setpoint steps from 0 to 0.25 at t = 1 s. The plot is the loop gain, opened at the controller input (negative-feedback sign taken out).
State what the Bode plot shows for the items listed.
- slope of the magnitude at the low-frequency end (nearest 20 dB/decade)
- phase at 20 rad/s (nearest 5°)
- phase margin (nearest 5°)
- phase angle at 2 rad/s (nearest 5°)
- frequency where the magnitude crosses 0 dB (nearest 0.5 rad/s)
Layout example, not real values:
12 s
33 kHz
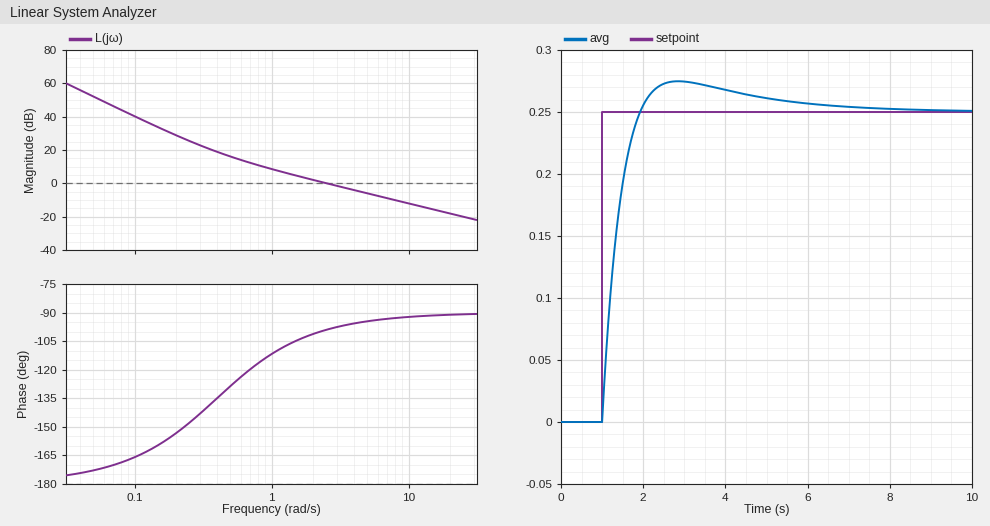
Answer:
-40 dB/decade
-90°
80°
-100°
2.5 rad/s
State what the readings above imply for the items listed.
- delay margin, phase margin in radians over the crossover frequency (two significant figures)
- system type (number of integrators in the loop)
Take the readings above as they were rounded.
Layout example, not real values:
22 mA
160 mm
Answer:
0.56 s
2
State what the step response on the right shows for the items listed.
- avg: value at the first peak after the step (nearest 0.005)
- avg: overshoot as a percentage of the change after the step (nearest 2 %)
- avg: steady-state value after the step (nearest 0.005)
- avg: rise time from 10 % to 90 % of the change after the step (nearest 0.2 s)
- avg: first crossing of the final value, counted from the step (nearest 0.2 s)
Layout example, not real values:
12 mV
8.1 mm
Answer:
0.275
10 %
0.250
0.6 s
1.0 s
